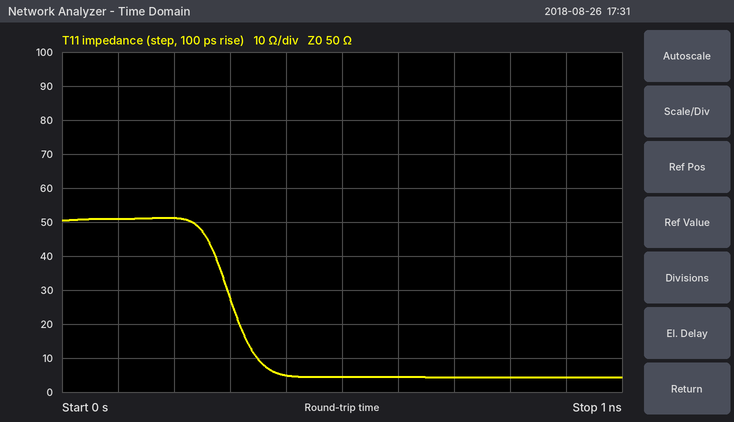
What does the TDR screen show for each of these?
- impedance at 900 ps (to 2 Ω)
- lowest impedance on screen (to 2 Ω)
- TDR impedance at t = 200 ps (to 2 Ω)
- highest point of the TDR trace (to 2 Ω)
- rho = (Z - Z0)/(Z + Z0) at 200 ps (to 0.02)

4 Ω
4 Ω
52 Ω
52 Ω
+0.02
